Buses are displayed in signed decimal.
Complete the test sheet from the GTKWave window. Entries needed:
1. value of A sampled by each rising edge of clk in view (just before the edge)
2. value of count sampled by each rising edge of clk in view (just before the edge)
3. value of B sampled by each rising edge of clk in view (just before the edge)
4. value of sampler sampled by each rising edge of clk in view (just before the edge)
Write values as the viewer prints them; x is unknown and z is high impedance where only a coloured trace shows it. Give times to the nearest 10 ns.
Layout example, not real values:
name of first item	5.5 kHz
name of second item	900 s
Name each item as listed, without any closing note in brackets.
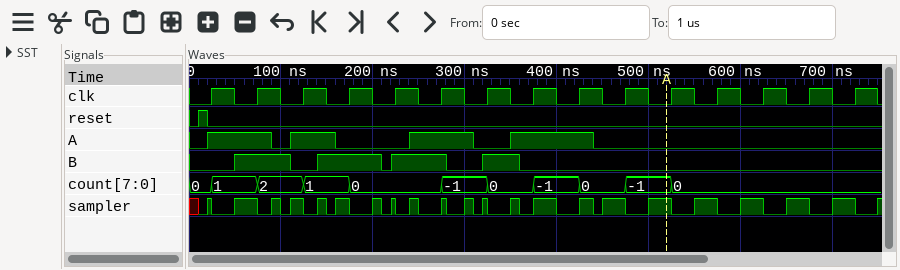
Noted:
value of A sampled by each rising edge of clk in view	1 1 1 0 0 1 0 1 1 0 0 0 0 0 0
value of count sampled by each rising edge of clk in view	0, 1, 2, 1, 0, 0, -1, 0, -1, 0, -1, 0, 0, 0, 0
value of B sampled by each rising edge of clk in view	0 1 0 1 1 1 1 0 0 0 0 0 0 0 0
value of sampler sampled by each rising edge of clk in view	1 1 1 1 1 0 1 0 0 1 1 1 1 1 1
